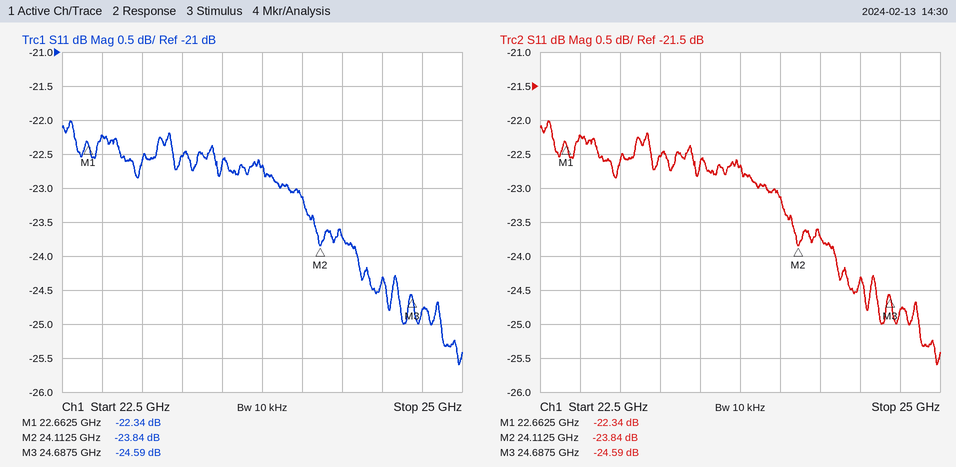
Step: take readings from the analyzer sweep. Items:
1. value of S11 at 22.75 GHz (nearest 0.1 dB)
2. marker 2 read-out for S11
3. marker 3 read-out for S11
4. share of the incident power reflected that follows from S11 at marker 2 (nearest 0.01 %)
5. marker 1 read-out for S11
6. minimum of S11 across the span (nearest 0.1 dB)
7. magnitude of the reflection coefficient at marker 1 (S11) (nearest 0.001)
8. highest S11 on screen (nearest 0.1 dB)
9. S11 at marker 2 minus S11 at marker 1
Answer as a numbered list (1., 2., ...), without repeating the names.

1. -22.2 dB
2. -23.84 dB
3. -24.59 dB
4. 0.41 %
5. -22.34 dB
6. -25.6 dB
7. 0.076
8. -22.0 dB
9. -1.50 dB
